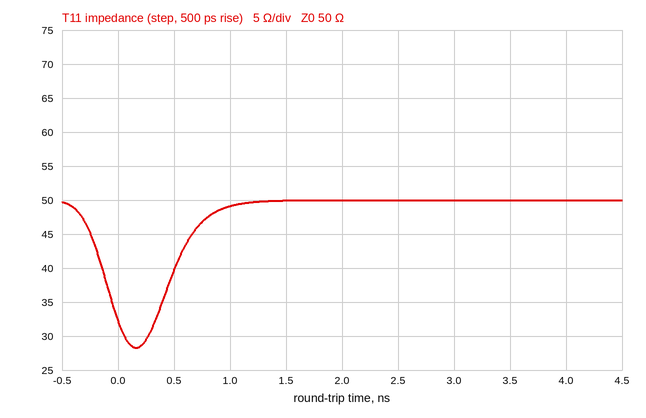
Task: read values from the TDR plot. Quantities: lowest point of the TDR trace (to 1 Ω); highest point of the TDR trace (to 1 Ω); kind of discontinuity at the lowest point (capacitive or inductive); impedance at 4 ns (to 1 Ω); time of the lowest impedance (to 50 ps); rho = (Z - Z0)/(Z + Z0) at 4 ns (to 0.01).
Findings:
28 Ω
50 Ω
capacitive
50 Ω
150 ps
0.00
